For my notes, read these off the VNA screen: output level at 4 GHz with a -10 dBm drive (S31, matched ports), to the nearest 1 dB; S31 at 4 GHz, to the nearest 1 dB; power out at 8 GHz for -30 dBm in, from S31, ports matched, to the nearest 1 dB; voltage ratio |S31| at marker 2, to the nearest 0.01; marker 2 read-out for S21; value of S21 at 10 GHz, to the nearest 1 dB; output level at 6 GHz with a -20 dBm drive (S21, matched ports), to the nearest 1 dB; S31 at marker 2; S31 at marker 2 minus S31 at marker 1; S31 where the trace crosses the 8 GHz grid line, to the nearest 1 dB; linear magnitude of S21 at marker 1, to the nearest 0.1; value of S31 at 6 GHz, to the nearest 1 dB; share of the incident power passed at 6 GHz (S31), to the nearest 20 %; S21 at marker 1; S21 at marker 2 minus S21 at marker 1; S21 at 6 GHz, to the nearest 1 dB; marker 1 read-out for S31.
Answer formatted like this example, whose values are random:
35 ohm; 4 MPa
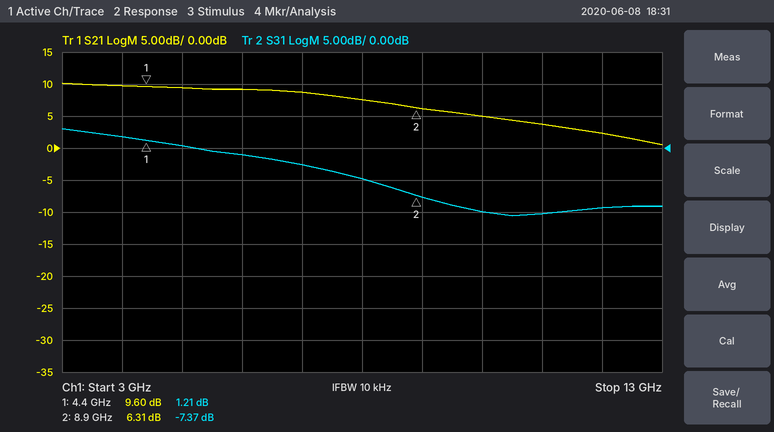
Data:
-8 dBm; 2 dB; -35 dBm; 0.43; 6.31 dB; 5 dB; -11 dBm; -7.37 dB; -8.58 dB; -5 dB; 3.0; -1 dB; 80 %; 9.60 dB; -3.29 dB; 9 dB; 1.21 dB
